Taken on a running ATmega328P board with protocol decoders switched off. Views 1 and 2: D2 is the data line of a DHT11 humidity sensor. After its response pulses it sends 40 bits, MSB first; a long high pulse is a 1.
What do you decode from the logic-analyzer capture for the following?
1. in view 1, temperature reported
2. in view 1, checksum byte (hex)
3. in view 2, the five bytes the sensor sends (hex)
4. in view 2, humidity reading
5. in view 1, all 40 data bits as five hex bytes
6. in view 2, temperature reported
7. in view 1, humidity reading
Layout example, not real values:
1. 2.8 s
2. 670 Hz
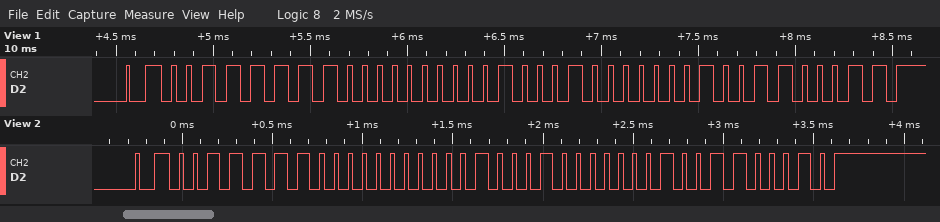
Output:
1. 34.2 °C
2. 0x63
3. 3E 00 22 02 62
4. 62 %
5. 3F 00 22 02 63
6. 34.2 °C
7. 63 %
